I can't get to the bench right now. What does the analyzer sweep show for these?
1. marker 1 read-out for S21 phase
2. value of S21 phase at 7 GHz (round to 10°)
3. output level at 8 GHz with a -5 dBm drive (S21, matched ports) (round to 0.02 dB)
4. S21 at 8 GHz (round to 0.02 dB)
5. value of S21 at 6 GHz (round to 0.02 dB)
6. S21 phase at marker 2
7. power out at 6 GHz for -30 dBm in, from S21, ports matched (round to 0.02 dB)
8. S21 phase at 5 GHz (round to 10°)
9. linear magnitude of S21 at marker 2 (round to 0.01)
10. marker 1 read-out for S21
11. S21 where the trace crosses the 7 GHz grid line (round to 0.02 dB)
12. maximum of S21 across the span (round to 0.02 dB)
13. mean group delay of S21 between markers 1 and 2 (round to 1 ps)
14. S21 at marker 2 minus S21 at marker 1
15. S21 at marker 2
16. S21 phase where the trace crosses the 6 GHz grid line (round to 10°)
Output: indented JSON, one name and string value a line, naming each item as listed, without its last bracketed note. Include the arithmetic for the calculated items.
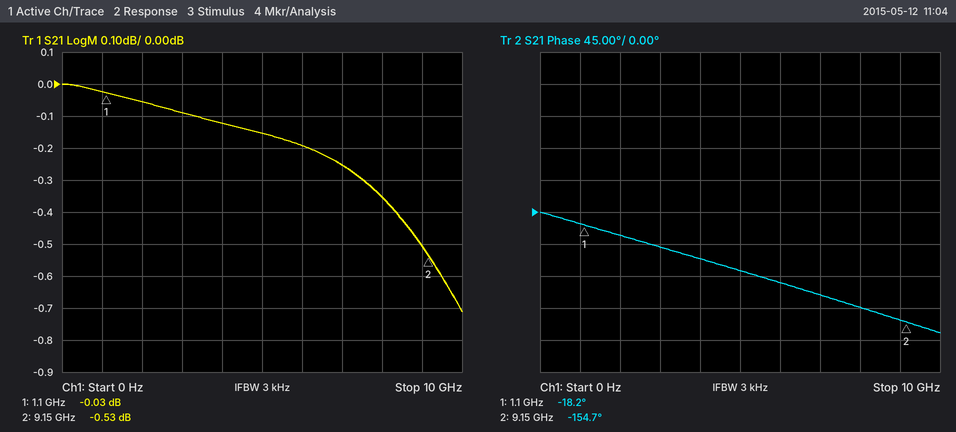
{
  "marker 1 read-out for S21 phase": "-18.2°",
  "value of S21 phase at 7 GHz": "-120°",
  "output level at 8 GHz with a -5 dBm drive (S21, matched ports)": "-5 dBm + (-0.36 dB) = -5.36 dBm",
  "S21 at 8 GHz": "-0.36 dB",
  "value of S21 at 6 GHz": "-0.20 dB",
  "S21 phase at marker 2": "-154.7°",
  "power out at 6 GHz for -30 dBm in, from S21, ports matched": "-30 dBm + (-0.20 dB) = -30.20 dBm",
  "S21 phase at 5 GHz": "-80°",
  "linear magnitude of S21 at marker 2": "10^(-0.53/20) ≈ 0.94",
  "marker 1 read-out for S21": "-0.03 dB",
  "S21 where the trace crosses the 7 GHz grid line": "-0.26 dB",
  "maximum of S21 across the span": "0.00 dB",
  "mean group delay of S21 between markers 1 and 2": "−(-154.7° − (-18.2°))/(360° × 8.05 GHz) ≈ 47 ps",
  "S21 at marker 2 minus S21 at marker 1": "-0.53 − (-0.03) = -0.50 dB",
  "S21 at marker 2": "-0.53 dB",
  "S21 phase where the trace crosses the 6 GHz grid line": "-100°"
}
